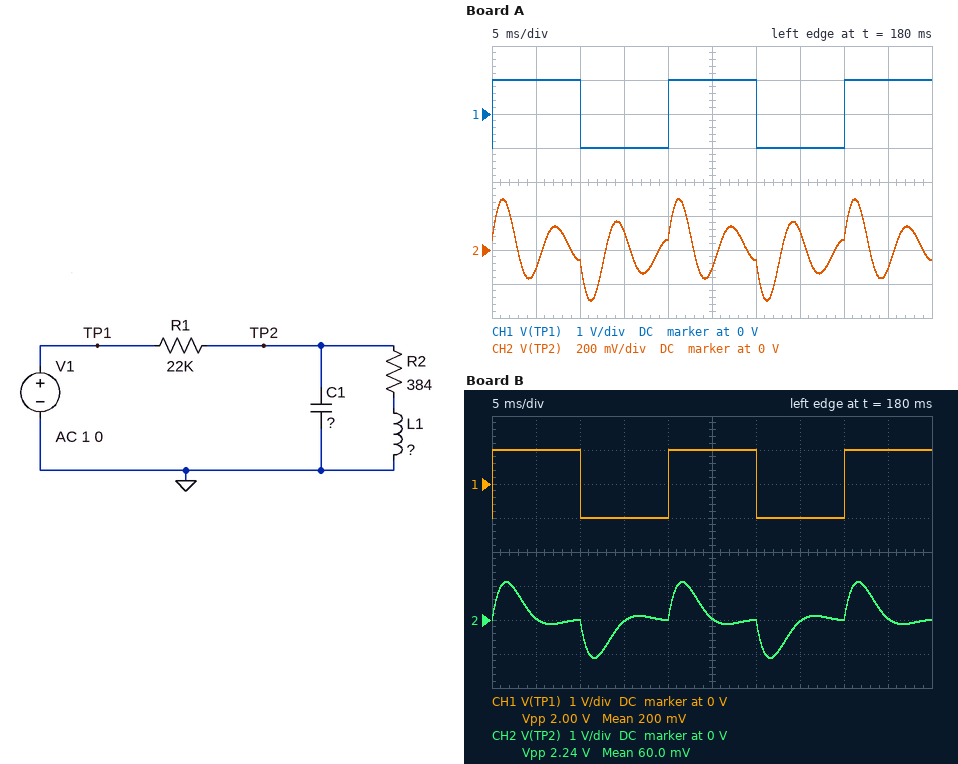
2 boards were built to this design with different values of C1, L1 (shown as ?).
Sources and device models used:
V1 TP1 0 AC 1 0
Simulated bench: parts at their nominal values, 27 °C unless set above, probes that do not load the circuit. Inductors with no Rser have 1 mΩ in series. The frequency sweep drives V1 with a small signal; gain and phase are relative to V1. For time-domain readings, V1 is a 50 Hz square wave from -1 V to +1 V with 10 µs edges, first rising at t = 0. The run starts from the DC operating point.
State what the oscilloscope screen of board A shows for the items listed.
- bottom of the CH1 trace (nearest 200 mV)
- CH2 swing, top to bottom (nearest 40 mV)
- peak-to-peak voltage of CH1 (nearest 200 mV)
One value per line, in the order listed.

-1.0 V
600 mV
2.0 V
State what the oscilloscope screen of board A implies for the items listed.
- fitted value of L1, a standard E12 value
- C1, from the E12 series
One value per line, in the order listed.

3.3 H
270 nF
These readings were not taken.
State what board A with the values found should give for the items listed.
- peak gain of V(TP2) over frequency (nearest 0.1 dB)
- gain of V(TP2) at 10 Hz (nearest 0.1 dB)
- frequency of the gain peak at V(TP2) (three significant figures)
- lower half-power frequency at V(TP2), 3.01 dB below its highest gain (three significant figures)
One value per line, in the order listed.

-4.5 dB
-34.2 dB
170 Hz
149 Hz
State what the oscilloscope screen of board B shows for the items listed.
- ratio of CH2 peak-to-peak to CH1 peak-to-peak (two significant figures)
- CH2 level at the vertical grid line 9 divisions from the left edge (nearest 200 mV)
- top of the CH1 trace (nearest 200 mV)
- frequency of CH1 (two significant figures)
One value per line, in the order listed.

1.1
0 V
1.0 V
50 Hz
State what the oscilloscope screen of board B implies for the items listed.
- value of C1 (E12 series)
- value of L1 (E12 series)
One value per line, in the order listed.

56 nF
33 H
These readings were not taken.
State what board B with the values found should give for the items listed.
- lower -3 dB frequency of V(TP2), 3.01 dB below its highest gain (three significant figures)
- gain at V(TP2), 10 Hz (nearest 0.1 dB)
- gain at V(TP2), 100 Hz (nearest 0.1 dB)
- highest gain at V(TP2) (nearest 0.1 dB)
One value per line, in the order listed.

69.5 Hz
-20.5 dB
-0.5 dB
-0.1 dB
